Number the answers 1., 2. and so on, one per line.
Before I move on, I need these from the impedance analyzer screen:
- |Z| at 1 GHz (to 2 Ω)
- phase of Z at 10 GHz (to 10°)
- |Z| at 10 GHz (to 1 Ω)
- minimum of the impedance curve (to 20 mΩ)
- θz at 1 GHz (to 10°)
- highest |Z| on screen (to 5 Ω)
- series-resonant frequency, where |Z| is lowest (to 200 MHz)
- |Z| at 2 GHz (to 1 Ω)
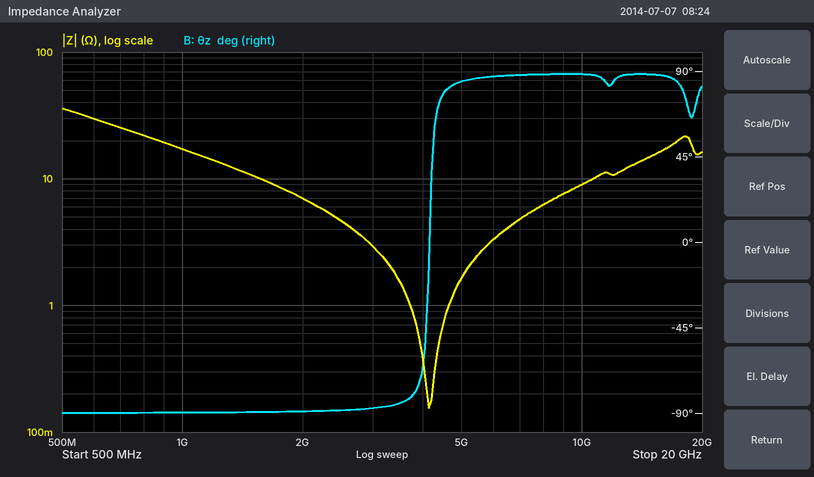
1. 18 Ω
2. 90°
3. 9 Ω
4. 160 mΩ
5. -90°
6. 35 Ω
7. 4.2 GHz
8. 7 Ω
